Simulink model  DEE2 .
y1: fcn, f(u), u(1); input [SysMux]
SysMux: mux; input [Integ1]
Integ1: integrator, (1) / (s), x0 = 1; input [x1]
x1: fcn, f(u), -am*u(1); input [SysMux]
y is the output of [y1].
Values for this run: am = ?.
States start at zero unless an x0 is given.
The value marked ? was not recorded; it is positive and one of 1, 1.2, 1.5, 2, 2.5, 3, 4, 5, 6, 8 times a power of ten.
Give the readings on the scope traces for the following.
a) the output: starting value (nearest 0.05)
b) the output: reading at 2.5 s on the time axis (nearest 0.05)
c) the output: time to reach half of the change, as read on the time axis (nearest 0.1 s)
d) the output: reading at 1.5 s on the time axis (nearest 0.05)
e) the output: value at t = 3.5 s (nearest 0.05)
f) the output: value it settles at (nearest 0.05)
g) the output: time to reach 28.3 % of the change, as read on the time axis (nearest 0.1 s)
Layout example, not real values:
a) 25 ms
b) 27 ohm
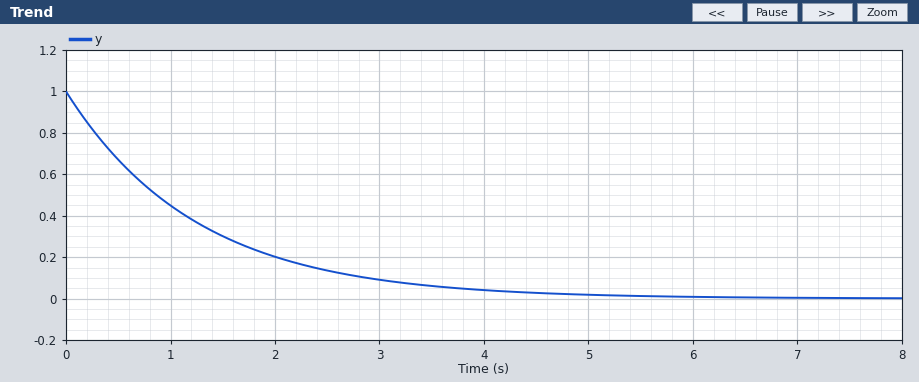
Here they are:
a) 1.00
b) 0.15
c) 0.9 s
d) 0.30
e) 0.05
f) 0.00
g) 0.4 s
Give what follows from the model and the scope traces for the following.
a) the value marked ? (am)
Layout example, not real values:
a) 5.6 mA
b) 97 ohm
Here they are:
a) 0.8
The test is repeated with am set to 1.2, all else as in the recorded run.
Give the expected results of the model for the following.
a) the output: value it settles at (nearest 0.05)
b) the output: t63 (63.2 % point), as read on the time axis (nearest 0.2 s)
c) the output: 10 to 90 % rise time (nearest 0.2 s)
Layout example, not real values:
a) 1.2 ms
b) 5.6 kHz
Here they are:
a) 0.00
b) 0.8 s
c) 1.8 s
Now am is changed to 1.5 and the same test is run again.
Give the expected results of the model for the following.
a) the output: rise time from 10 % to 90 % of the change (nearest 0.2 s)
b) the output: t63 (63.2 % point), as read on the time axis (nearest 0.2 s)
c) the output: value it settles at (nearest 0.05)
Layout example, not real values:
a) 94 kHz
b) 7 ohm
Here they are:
a) 1.4 s
b) 0.6 s
c) 0.00
